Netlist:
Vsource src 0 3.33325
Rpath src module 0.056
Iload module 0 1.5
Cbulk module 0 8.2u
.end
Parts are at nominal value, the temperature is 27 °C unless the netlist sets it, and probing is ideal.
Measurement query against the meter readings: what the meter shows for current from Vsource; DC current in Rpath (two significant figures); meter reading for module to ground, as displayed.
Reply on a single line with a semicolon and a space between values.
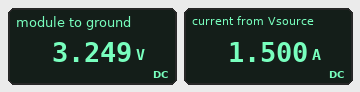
1.500 A; 1.5 A; 3.249 V
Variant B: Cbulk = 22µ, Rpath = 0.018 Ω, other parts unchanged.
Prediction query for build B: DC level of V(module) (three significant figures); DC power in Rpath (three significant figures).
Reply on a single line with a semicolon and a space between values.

3.31 V; 40.5 mW
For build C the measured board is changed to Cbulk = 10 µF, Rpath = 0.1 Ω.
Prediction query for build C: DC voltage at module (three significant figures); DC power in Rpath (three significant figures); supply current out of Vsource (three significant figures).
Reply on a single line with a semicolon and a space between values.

3.18 V; 225 mW; 1.50 A
